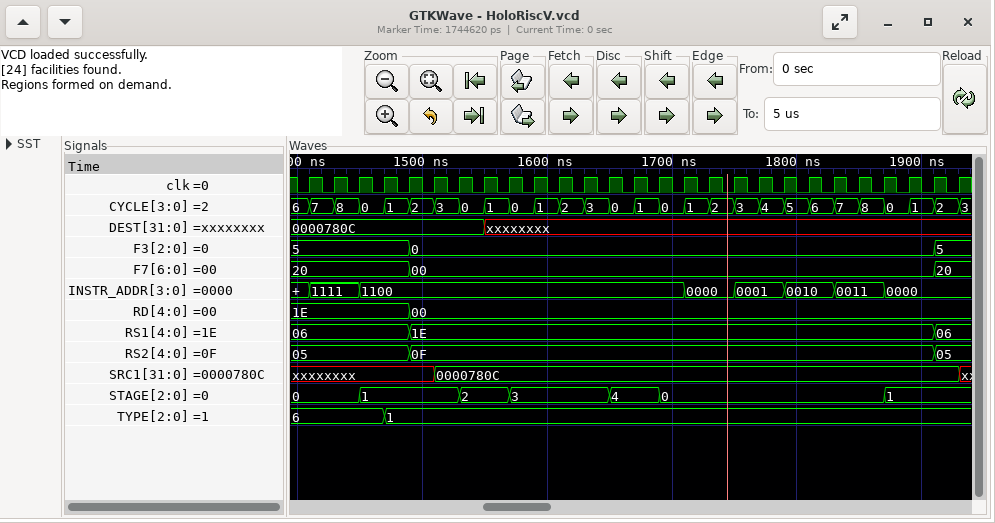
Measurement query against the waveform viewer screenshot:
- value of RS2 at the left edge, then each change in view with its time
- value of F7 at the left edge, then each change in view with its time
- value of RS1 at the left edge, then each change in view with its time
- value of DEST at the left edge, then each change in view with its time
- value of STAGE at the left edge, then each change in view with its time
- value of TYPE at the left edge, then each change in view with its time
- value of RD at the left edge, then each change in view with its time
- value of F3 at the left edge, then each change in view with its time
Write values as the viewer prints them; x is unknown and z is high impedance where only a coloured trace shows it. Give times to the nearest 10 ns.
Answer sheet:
05, 0F at 1490 ns, 05 at 1910 ns
20, 00 at 1490 ns, 20 at 1910 ns
06, 1E at 1490 ns, 06 at 1910 ns
0000780C, xxxxxxxx at 1550 ns
0, 1 at 1450 ns, 2 at 1530 ns, 3 at 1570 ns, 4 at 1650 ns, 0 at 1690 ns, 1 at 1870 ns
6, 1 at 1470 ns
1E, 00 at 1490 ns
5, 0 at 1490 ns, 5 at 1910 ns
